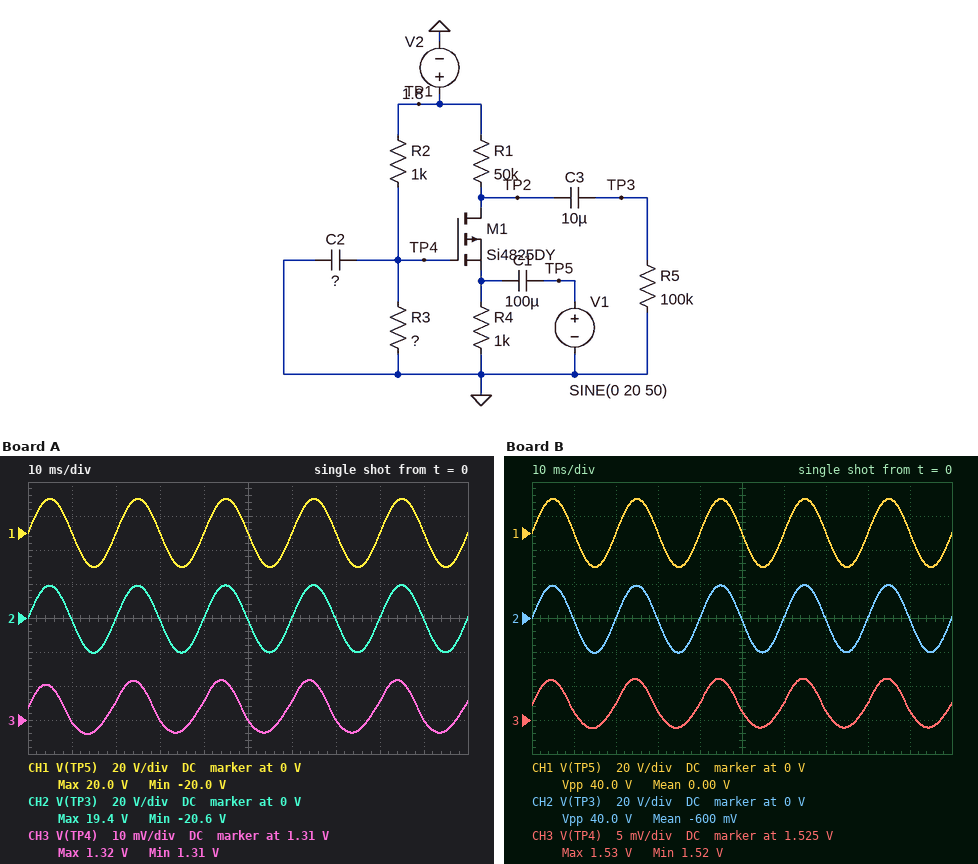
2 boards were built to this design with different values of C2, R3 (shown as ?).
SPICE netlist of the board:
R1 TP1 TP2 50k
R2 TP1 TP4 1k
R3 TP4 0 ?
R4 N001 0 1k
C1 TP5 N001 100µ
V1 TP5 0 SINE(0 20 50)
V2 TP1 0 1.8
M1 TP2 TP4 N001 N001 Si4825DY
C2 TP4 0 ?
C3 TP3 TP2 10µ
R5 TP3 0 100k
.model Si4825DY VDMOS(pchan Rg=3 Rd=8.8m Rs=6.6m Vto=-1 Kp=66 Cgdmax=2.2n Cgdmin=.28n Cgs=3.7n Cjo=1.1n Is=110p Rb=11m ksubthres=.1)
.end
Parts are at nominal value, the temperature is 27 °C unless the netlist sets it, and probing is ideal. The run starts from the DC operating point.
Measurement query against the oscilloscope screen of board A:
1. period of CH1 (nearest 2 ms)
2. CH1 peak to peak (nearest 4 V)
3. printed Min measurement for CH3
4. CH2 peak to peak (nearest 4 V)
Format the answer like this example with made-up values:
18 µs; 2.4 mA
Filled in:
20 ms; 40 V; 1.31 V; 40 V
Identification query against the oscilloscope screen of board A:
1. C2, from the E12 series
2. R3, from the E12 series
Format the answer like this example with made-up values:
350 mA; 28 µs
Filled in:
12 µF; 2.7 kΩ
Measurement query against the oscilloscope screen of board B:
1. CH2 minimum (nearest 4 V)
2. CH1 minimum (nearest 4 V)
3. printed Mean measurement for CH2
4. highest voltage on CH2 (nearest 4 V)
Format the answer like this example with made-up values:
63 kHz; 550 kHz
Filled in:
-20 V; -20 V; -600 mV; 20 V
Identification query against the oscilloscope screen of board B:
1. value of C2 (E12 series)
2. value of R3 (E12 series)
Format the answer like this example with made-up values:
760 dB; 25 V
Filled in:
27 µF; 5.6 kΩ
